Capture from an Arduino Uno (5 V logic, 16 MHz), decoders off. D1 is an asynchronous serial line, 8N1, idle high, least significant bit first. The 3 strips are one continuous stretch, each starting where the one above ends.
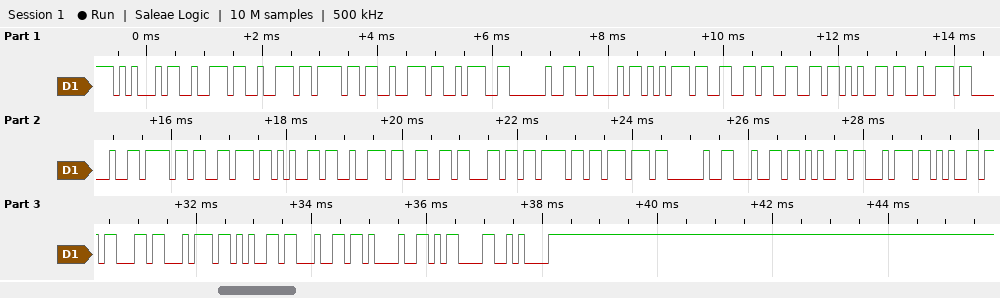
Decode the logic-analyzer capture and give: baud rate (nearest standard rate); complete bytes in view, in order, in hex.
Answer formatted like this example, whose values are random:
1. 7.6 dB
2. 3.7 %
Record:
1. 9600 baud
2. 0x45 0x72 0x72 0x6F 0x72 0x3A 0x20 0x42 0x75 0x66 0x66 0x65 0x72 0x20 0x6F 0x76 0x65 0x72 0x66 0x6C 0x6F 0x77 0x20 0x64 0x65 0x74 0x65 0x63 0x74 0x65 0x64 0x21 0x0D 0x0A
